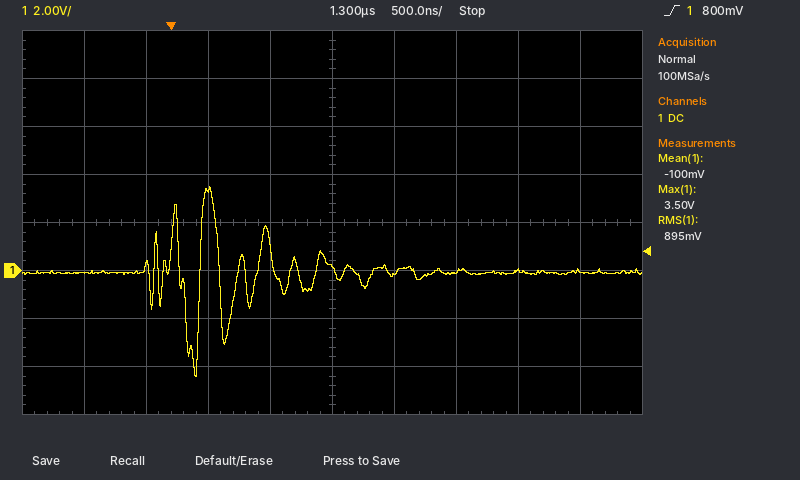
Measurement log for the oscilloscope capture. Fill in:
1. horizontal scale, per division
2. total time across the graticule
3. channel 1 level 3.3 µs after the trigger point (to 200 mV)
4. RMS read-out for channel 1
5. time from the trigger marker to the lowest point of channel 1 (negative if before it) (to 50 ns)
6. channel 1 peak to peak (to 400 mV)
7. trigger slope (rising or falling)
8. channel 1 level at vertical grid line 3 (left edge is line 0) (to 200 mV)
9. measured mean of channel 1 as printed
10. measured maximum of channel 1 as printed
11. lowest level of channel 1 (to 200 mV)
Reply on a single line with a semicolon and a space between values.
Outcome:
500 ns; 5 µs; 0.0 V; 895 mV; +200 ns; 8.0 V; rising; 3.4 V; -100 mV; 3.50 V; -4.4 V
